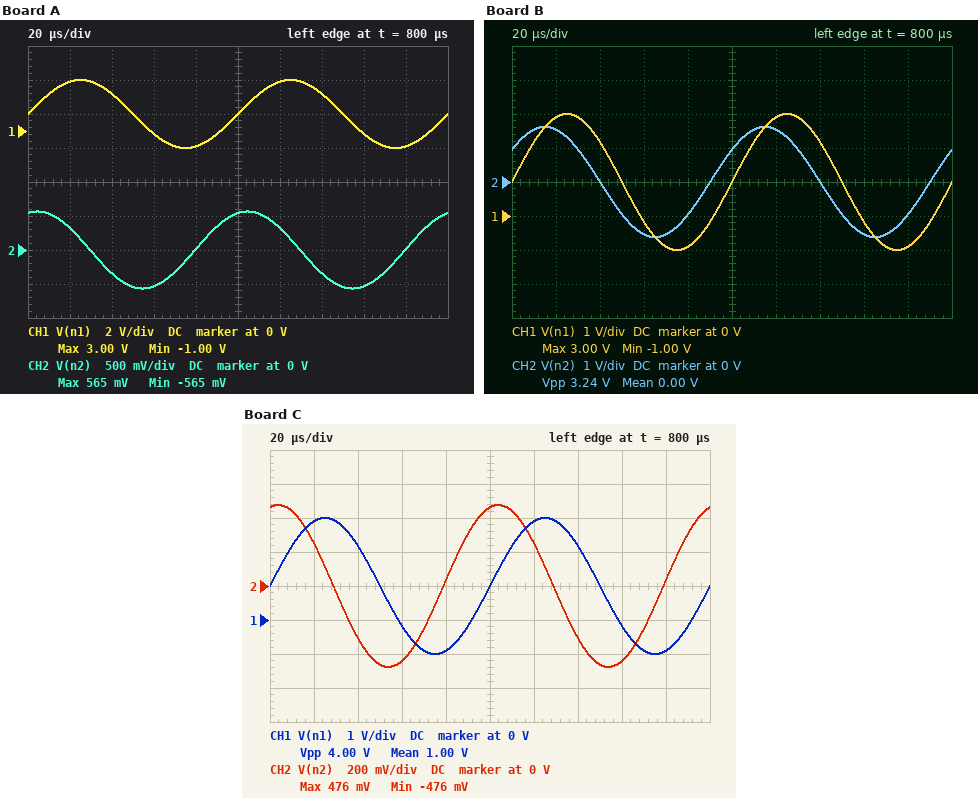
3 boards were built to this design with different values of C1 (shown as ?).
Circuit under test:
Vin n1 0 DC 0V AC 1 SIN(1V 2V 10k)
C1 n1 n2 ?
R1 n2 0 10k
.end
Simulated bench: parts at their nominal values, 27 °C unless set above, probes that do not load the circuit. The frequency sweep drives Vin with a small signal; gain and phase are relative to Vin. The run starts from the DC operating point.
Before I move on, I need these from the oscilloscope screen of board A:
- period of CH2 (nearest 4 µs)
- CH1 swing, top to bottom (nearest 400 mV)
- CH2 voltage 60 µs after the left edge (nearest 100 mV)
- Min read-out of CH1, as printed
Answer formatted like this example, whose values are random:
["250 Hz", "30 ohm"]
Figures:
["100 µs", "4.0 V", "-500 mV", "-1.00 V"]
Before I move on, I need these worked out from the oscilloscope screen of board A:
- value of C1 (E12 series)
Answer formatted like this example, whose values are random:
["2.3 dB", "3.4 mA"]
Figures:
["470 pF"]
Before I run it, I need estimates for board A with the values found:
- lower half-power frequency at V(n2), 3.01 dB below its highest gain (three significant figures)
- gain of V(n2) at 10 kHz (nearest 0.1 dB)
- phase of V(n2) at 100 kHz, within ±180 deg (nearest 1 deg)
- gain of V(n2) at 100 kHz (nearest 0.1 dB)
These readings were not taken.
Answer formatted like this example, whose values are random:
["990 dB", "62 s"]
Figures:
["33.9 kHz", "-11.0 dB", "19 deg", "-0.5 dB"]
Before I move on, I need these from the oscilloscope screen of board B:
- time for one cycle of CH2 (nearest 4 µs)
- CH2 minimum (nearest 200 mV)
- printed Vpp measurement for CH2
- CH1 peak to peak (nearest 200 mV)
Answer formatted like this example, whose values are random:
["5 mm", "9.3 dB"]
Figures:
["100 µs", "-1.6 V", "3.24 V", "4.0 V"]
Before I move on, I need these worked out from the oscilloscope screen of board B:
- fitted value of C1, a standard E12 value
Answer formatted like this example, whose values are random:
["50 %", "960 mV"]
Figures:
["2.2 nF"]
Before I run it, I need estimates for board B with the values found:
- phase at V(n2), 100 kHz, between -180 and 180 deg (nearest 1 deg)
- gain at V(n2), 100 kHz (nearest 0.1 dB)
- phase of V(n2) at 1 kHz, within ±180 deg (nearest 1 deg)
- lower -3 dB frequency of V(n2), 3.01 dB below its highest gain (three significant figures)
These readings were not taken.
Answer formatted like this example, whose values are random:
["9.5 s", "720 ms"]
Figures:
["4 deg", "0 dB", "82 deg", "7.23 kHz"]
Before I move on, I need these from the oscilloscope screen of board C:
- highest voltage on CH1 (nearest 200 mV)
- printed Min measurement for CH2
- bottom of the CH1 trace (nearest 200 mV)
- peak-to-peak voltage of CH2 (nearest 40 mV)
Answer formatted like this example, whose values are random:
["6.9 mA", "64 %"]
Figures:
["3.0 V", "-476 mV", "-1.0 V", "960 mV"]
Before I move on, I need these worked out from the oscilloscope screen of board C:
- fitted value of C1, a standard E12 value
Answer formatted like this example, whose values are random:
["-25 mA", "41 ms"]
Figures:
["390 pF"]
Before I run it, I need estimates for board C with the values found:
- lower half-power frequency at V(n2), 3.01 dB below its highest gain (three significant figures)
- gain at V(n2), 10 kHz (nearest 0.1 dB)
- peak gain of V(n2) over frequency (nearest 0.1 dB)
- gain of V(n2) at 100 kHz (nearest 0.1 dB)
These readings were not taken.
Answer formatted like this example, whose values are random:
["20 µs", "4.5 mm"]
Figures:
["40.8 kHz", "-12.5 dB", "0 dB", "-0.7 dB"]
